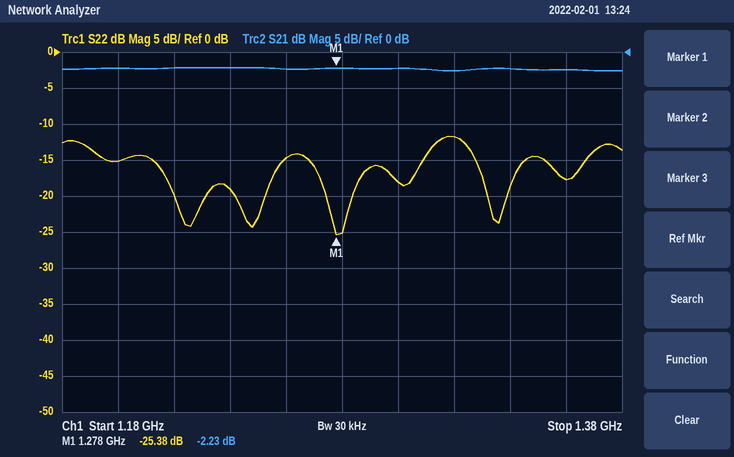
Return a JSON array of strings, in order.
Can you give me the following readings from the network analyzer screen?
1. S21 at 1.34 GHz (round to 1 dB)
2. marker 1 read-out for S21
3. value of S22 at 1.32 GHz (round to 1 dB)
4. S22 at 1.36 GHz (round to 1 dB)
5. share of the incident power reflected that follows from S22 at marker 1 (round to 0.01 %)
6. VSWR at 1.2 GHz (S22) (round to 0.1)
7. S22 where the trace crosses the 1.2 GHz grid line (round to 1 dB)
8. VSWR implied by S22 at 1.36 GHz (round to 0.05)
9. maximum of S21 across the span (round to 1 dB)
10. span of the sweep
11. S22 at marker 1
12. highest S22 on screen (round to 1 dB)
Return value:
["-2 dB", "-2.23 dB", "-12 dB", "-18 dB", "0.29 %", "1.4", "-15 dB", "1.30", "-2 dB", "200 MHz", "-25.38 dB", "-12 dB"]
